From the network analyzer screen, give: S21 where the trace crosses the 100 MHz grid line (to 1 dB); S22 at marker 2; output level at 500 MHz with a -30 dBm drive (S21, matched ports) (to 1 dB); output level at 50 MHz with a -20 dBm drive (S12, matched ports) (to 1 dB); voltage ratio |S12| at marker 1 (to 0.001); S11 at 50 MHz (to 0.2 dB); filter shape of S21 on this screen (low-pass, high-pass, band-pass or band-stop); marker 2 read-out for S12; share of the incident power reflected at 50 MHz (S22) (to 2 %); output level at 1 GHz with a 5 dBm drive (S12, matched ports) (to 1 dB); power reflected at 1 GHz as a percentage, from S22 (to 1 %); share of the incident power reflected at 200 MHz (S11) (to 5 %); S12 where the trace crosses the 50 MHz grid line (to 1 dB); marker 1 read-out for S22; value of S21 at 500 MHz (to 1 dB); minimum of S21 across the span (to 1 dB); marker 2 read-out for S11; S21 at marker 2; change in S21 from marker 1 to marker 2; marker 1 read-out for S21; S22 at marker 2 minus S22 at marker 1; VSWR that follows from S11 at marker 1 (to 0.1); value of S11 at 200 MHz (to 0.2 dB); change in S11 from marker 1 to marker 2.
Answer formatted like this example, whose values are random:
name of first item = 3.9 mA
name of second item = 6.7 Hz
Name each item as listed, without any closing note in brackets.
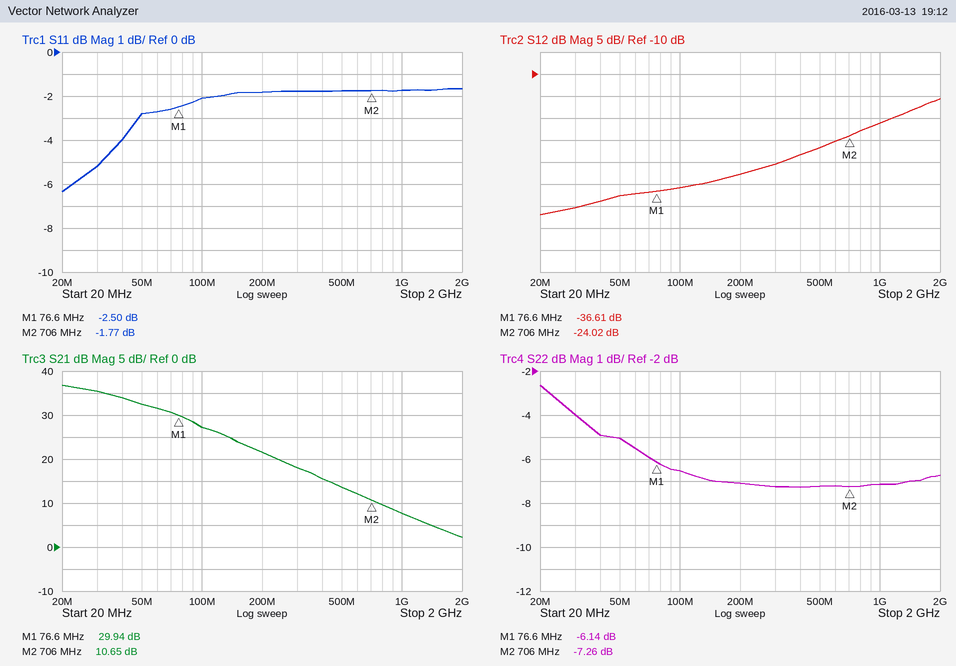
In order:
S21 where the trace crosses the 100 MHz grid line = 27 dB
S22 at marker 2 = -7.26 dB
output level at 500 MHz with a -30 dBm drive (S21, matched ports) = -16 dBm
output level at 50 MHz with a -20 dBm drive (S12, matched ports) = -58 dBm
voltage ratio |S12| at marker 1 = 0.015
S11 at 50 MHz = -2.8 dB
filter shape of S21 on this screen = low-pass
marker 2 read-out for S12 = -24.02 dB
share of the incident power reflected at 50 MHz (S22) = 32 %
output level at 1 GHz with a 5 dBm drive (S12, matched ports) = -16 dBm
power reflected at 1 GHz as a percentage, from S22 = 19 %
share of the incident power reflected at 200 MHz (S11) = 65 %
S12 where the trace crosses the 50 MHz grid line = -38 dB
marker 1 read-out for S22 = -6.14 dB
value of S21 at 500 MHz = 14 dB
minimum of S21 across the span = 2 dB
marker 2 read-out for S11 = -1.77 dB
S21 at marker 2 = 10.65 dB
change in S21 from marker 1 to marker 2 = -19.29 dB
marker 1 read-out for S21 = 29.94 dB
S22 at marker 2 minus S22 at marker 1 = -1.12 dB
VSWR that follows from S11 at marker 1 = 7.0
value of S11 at 200 MHz = -1.8 dB
change in S11 from marker 1 to marker 2 = 0.73 dB
